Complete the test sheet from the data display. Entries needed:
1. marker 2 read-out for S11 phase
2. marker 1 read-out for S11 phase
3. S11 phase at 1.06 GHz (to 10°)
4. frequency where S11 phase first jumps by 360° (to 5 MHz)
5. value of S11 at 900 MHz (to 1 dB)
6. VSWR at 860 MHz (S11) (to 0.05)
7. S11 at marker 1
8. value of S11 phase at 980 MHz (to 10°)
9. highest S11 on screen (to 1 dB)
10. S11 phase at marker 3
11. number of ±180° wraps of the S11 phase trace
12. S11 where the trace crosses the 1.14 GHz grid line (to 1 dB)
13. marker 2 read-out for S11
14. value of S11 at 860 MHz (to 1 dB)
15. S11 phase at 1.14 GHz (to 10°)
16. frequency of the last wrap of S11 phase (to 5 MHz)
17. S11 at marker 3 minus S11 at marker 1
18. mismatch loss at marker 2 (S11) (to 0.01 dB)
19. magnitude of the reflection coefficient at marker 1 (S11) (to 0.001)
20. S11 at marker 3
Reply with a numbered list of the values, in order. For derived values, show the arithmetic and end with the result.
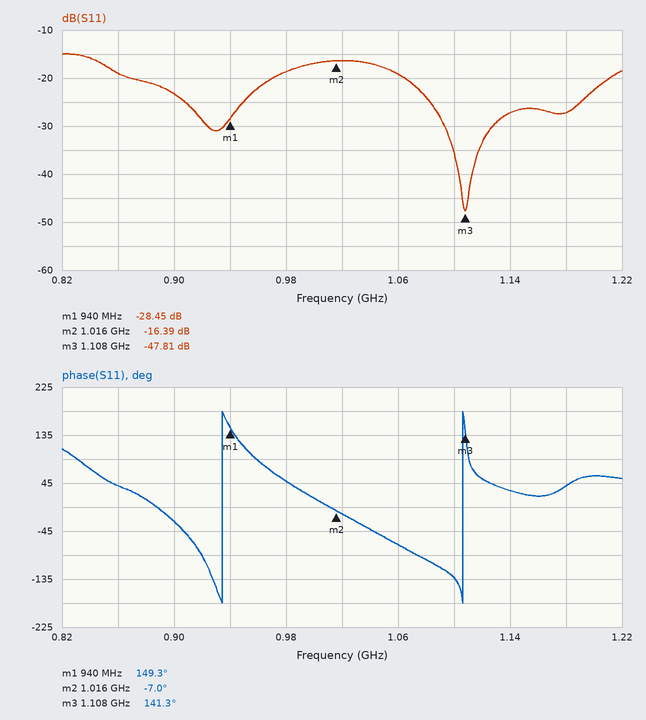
1. -7.0°
2. 149.3°
3. -70°
4. 935 MHz
5. -23 dB
6. |Γ| = 10^(-19/20) = 0.1122; VSWR = (1 + 0.1122)/(1 − 0.1122) ≈ 1.25
7. -28.45 dB
8. 50°
9. -15 dB
10. 141.3°
11. 2
12. -27 dB
13. -16.39 dB
14. -19 dB
15. 30°
16. 1.105 GHz
17. -47.81 − (-28.45) = -19.36 dB
18. −10 log10(1 − 10^(-16.39/10)) ≈ 0.10 dB
19. 10^(-28.45/20) ≈ 0.038
20. -47.81 dB
